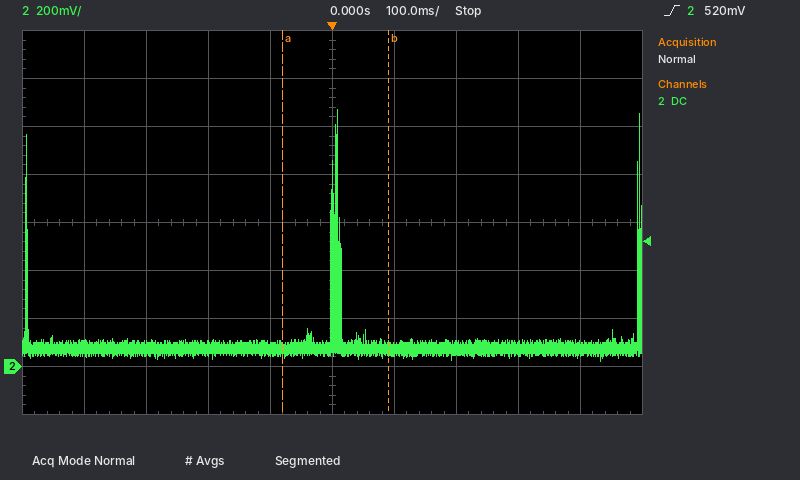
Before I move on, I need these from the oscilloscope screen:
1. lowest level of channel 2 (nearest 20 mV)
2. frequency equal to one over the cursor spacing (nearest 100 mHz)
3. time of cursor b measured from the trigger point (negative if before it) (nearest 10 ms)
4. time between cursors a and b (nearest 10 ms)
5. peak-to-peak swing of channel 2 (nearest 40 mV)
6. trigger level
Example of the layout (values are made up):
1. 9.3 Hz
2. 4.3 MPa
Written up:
1. 20 mV
2. 5.9 Hz
3. +90 ms
4. 170 ms
5. 1.04 V
6. 520 mV
